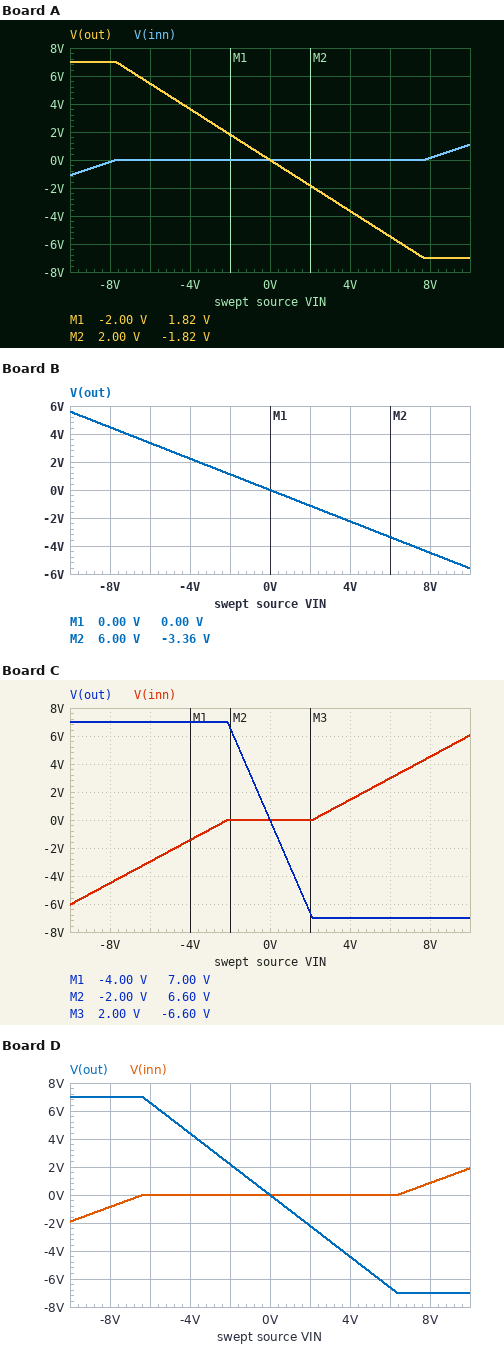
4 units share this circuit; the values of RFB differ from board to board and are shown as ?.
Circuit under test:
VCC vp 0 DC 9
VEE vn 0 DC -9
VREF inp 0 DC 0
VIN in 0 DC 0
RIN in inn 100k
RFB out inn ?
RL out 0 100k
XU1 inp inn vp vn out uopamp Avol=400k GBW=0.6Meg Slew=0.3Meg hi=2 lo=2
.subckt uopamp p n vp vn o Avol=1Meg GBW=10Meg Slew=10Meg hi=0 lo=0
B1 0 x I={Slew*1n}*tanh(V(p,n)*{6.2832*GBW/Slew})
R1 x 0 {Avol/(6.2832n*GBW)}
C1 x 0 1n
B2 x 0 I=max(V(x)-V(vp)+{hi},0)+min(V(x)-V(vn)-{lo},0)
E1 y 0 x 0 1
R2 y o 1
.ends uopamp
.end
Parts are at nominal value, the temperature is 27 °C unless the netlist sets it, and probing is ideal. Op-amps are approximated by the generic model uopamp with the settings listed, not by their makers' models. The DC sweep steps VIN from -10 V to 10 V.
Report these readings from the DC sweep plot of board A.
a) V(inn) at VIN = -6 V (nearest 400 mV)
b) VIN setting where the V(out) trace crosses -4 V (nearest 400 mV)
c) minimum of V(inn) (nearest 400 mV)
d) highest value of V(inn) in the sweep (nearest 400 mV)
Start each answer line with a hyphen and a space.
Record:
- 0 V
- 4.4 V
- -1.2 V
- 1.2 V
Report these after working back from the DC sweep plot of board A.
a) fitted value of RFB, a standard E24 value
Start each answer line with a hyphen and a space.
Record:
- 91 kΩ
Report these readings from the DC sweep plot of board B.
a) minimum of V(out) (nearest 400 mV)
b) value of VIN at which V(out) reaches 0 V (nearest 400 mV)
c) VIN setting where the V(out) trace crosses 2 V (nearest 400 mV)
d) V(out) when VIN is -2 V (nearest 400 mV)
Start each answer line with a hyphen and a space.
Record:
- -5.6 V
- 0 V
- -3.6 V
- 1.2 V
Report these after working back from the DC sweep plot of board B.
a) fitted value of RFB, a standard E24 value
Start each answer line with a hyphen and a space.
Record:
- 56 kΩ
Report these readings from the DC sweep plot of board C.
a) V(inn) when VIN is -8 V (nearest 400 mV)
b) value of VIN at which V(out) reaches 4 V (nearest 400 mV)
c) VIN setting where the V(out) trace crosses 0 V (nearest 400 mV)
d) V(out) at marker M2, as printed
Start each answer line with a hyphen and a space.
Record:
- -4.4 V
- -1.2 V
- 0 V
- 6.60 V
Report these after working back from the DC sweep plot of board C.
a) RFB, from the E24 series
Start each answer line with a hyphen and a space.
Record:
- 330 kΩ
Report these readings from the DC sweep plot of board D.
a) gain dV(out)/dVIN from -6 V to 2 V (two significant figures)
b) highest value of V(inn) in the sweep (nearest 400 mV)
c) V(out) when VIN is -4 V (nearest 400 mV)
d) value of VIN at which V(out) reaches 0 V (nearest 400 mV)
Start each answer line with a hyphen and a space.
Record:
- -1.1 V/V
- 2.0 V
- 4.4 V
- 0 V
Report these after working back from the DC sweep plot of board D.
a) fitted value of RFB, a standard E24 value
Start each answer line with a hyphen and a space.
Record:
- 110 kΩ
